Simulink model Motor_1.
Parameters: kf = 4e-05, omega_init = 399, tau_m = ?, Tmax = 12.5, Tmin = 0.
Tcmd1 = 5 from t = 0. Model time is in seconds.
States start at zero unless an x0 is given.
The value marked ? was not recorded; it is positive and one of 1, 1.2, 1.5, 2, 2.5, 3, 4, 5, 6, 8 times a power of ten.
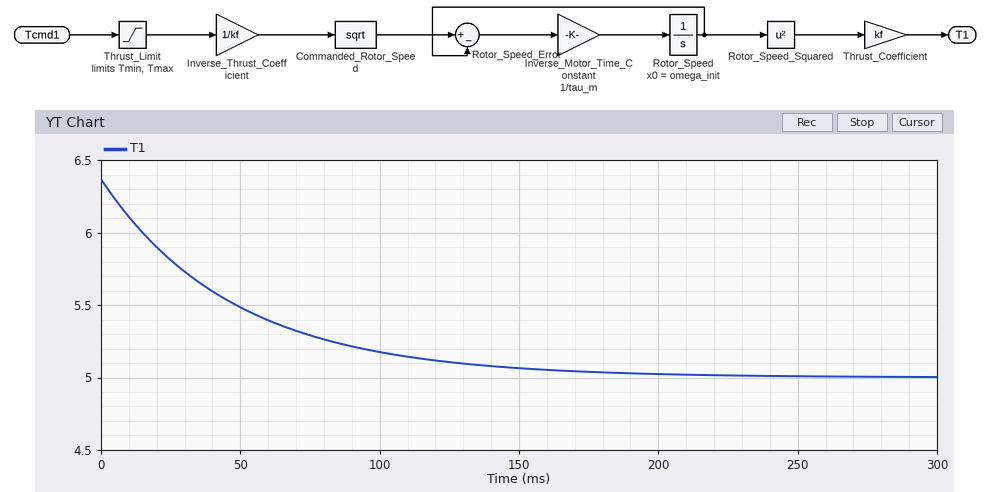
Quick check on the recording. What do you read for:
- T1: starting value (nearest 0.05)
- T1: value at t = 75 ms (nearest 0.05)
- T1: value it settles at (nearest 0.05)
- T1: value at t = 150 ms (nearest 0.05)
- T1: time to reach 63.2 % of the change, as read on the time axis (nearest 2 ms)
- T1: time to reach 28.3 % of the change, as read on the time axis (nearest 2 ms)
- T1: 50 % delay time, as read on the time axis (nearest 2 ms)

6.35
5.30
5.00
5.05
48 ms
16 ms
34 ms
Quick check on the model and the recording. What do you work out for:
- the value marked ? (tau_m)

0.05
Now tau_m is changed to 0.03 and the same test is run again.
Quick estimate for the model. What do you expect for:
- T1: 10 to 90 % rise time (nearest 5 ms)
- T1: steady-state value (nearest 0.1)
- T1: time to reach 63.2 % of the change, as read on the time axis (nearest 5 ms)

65 ms
5.0
30 ms
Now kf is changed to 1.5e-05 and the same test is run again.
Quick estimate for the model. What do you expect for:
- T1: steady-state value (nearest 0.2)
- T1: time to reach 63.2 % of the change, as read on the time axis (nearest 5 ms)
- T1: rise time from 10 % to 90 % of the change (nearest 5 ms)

5.0
55 ms
115 ms
